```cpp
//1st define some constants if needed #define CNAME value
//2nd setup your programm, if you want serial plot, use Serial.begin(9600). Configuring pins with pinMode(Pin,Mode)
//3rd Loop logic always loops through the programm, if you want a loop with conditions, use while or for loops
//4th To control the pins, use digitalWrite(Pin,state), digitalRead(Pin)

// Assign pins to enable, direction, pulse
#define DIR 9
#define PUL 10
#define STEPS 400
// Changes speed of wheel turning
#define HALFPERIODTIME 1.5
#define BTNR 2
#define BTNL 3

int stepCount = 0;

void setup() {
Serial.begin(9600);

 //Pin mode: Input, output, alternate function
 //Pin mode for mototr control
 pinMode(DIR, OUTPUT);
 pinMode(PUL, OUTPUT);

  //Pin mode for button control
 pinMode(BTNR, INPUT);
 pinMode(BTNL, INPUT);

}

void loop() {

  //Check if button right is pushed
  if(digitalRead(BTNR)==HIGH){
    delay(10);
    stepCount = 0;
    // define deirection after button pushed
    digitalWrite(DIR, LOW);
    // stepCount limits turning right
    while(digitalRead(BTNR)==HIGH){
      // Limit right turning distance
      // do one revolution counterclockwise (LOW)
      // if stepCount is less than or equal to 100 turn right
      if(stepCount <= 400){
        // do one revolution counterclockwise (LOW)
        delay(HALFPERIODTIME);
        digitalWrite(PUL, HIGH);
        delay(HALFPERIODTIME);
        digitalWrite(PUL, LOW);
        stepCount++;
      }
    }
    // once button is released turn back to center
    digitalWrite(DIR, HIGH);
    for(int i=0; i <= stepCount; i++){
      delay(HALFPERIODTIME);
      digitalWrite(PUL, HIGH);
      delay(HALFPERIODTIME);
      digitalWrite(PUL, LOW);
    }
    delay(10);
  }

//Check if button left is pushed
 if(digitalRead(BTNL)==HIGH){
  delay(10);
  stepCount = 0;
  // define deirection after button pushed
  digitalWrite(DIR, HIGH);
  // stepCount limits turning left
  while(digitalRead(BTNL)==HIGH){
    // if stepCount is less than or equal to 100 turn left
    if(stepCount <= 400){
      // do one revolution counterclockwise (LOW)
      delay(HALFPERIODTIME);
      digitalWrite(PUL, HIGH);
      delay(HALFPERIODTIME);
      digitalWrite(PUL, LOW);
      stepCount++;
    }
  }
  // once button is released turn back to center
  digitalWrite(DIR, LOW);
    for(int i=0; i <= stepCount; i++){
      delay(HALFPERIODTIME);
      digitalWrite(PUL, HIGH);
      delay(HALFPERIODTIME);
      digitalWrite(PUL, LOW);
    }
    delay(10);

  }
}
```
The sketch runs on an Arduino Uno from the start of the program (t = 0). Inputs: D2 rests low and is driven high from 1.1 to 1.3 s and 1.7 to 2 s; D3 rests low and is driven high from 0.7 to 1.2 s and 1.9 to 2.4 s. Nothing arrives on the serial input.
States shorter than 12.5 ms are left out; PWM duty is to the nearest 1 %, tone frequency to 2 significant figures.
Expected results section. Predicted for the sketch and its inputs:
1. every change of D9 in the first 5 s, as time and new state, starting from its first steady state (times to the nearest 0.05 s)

0 s low; 0.7 s high; 1.2 s low; 2 s high; 2.4 s low
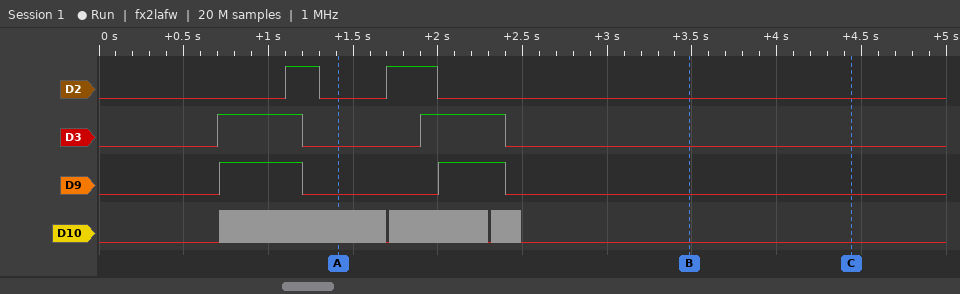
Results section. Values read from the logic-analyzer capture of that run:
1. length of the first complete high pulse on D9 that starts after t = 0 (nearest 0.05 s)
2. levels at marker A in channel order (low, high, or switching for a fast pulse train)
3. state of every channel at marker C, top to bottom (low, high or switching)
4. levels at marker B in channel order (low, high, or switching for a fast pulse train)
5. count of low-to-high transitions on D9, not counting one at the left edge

0.50 s
D2 low, D3 low, D9 low, D10 switching
D2 low, D3 low, D9 low, D10 low
D2 low, D3 low, D9 low, D10 low
2
